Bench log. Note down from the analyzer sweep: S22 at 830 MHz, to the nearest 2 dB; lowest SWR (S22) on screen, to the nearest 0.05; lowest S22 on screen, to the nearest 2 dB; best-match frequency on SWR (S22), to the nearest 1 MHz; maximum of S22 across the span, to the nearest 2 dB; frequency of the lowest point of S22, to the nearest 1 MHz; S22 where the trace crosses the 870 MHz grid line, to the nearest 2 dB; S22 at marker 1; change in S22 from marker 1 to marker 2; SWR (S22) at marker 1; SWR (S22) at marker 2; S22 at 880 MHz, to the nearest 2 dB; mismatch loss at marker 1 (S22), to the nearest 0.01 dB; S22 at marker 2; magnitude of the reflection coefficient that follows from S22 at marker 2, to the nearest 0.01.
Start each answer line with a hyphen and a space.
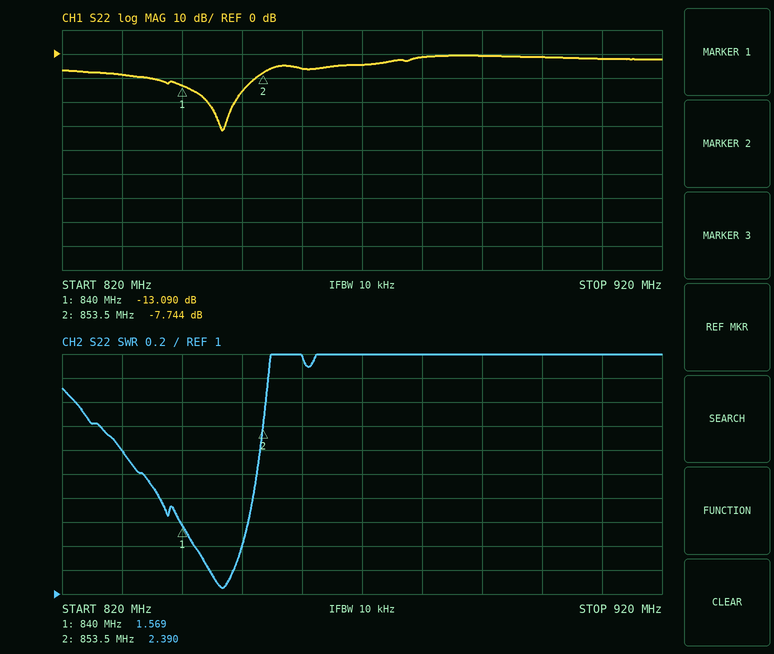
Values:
- -8 dB
- 1.05
- -32 dB
- 847 MHz
- 0 dB
- 847 MHz
- -4 dB
- -13.090 dB
- 5.346 dB
- 1.569
- 2.390
- -2 dB
- 0.22 dB
- -7.744 dB
- 0.41
